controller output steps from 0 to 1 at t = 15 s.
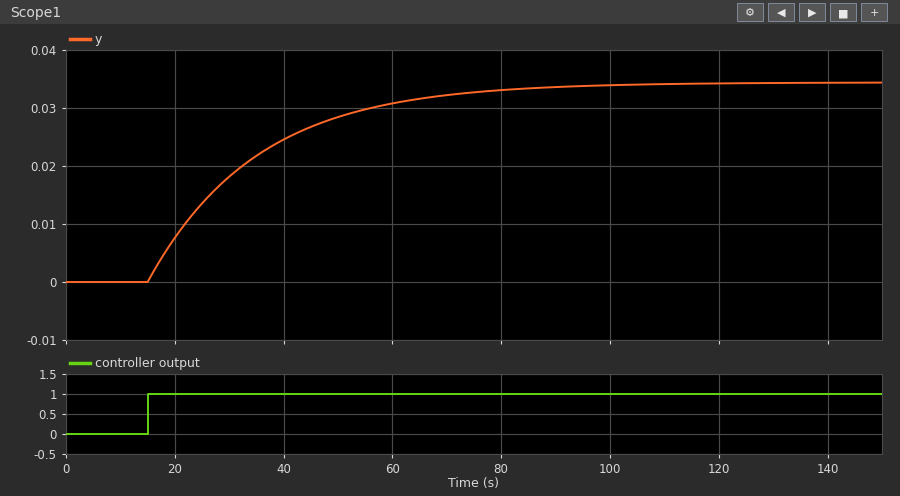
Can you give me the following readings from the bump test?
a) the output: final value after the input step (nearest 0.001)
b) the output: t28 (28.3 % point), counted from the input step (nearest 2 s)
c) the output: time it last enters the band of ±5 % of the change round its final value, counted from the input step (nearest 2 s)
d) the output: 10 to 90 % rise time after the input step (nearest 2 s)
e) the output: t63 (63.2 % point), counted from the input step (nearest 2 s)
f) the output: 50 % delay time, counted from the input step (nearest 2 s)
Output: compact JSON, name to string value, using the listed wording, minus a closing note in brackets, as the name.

{"the output: final value after the input step": "0.034", "the output: t28 (28.3 % point), counted from the input step": "6 s", "the output: time it last enters the band of ±5 % of the change round its final value, counted from the input step": "60 s", "the output: 10 to 90 % rise time after the input step": "44 s", "the output: t63 (63.2 % point), counted from the input step": "20 s", "the output: 50 % delay time, counted from the input step": "14 s"}
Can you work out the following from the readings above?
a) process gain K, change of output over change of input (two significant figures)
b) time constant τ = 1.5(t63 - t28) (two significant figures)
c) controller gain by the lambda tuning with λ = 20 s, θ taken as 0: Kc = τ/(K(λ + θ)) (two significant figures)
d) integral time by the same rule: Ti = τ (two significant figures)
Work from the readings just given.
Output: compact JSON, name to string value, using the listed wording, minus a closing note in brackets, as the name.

{"process gain K, change of output over change of input": "0.034", "time constant τ = 1.5(t63 - t28)": "21 s", "controller gain by the lambda tuning with λ = 20 s, θ taken as 0: Kc = τ/(K(λ + θ))": "31", "integral time by the same rule: Ti = τ": "21 s"}
